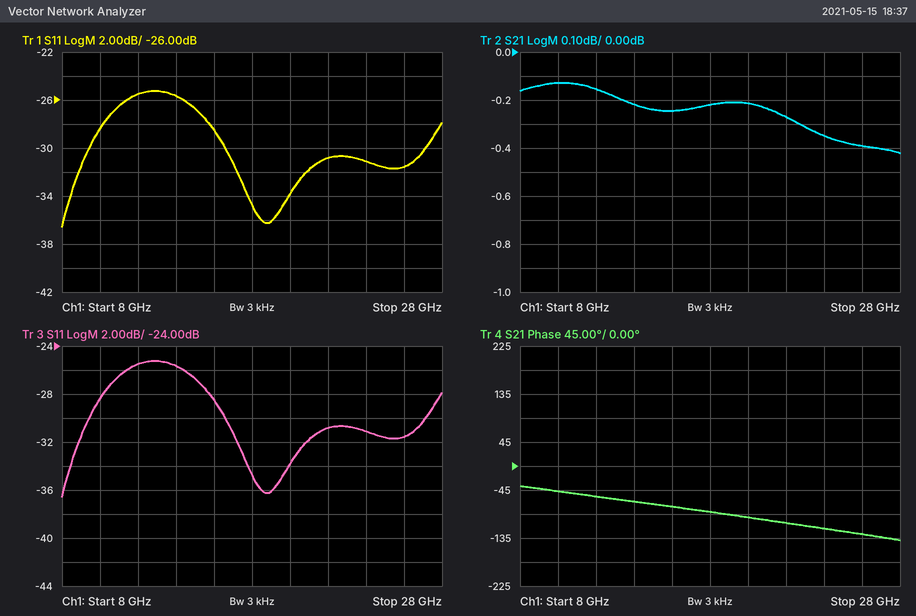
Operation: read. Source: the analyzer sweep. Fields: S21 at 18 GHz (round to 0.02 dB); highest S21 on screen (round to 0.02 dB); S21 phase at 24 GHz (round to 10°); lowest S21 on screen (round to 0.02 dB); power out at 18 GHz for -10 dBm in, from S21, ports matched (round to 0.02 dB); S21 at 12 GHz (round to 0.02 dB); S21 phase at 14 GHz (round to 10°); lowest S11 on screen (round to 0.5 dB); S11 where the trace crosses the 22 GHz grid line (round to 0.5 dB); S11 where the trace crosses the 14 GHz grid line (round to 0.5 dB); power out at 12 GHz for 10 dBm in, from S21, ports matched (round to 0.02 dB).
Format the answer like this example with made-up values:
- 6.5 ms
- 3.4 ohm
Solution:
- -0.22 dB
- -0.12 dB
- -120°
- -0.42 dB
- -10.22 dBm
- -0.16 dB
- -70°
- -36.5 dB
- -31.0 dB
- -25.5 dB
- 9.84 dBm
